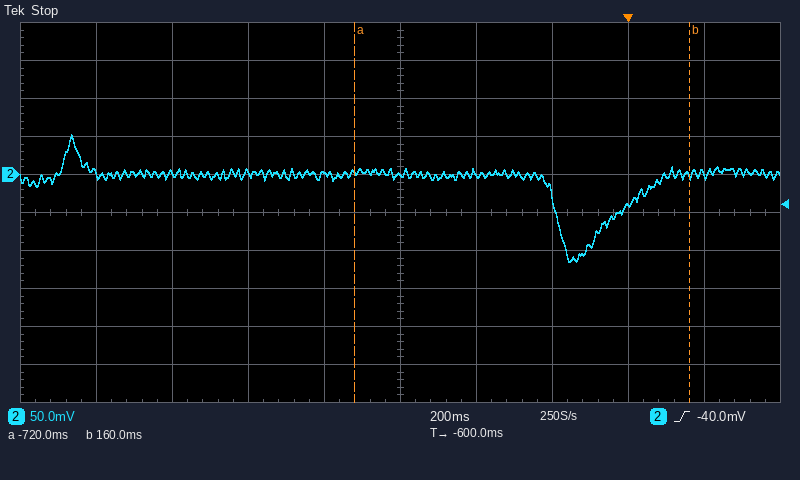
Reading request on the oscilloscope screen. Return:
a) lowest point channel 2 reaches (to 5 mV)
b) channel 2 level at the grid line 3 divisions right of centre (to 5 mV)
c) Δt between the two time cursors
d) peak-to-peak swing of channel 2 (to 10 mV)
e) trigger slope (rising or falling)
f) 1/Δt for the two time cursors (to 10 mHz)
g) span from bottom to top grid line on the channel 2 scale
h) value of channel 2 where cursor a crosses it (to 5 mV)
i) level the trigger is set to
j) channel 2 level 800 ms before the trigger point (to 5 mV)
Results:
-115 mV
-40 mV
880 ms
170 mV
rising
1.14 Hz
500 mV
5 mV
-40.0 mV
0 mV
